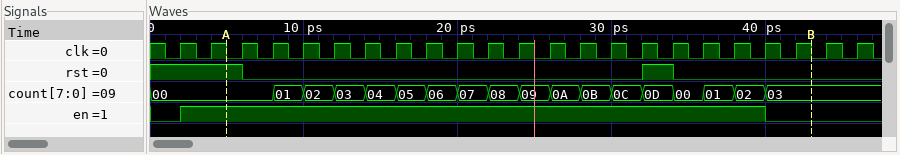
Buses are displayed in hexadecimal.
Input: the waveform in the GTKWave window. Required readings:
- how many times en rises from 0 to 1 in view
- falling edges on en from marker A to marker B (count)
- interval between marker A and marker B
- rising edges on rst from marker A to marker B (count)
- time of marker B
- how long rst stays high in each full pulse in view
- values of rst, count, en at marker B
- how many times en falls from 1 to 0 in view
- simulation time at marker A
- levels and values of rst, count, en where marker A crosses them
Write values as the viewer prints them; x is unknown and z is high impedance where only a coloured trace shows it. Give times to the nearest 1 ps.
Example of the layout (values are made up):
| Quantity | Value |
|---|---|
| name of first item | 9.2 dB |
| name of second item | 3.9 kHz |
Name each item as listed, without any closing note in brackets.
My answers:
| Quantity | Value |
|---|---|
| how many times en rises from 0 to 1 in view | 1 |
| falling edges on en from marker A to marker B | 1 |
| interval between marker A and marker B | 38 ps |
| rising edges on rst from marker A to marker B | 1 |
| time of marker B | 43 ps |
| how long rst stays high in each full pulse in view | 2 ps |
| values of rst, count, en at marker B | rst=0, count=03, en=0 |
| how many times en falls from 1 to 0 in view | 1 |
| simulation time at marker A | 5 ps |
| levels and values of rst, count, en where marker A crosses them | rst=1, count=00, en=1 |
